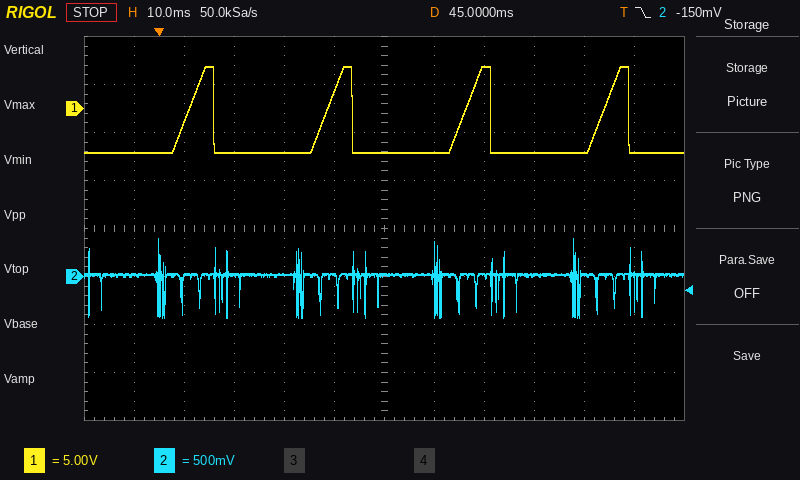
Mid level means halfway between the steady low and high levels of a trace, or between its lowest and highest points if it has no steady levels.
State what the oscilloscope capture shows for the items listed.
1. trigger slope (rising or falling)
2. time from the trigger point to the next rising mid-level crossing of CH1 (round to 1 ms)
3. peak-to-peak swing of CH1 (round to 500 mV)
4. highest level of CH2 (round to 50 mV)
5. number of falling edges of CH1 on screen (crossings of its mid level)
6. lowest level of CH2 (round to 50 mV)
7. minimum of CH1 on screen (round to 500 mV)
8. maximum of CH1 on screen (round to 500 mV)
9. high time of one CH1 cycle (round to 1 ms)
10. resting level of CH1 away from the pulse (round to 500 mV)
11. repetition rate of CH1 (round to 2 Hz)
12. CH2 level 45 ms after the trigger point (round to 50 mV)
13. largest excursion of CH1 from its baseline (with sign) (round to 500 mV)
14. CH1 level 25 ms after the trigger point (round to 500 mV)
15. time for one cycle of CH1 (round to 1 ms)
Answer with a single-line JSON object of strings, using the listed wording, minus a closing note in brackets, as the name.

{"trigger slope": "falling", "time from the trigger point to the next rising mid-level crossing of CH1": "6 ms", "peak-to-peak swing of CH1": "9.0 V", "highest level of CH2": "400 mV", "number of falling edges of CH1 on screen": "4", "lowest level of CH2": "-450 mV", "minimum of CH1 on screen": "-4.5 V", "maximum of CH1 on screen": "4.5 V", "high time of one CH1 cycle": "5 ms", "resting level of CH1 away from the pulse": "-4.5 V", "repetition rate of CH1": "36 Hz", "CH2 level 45 ms after the trigger point": "0 mV", "largest excursion of CH1 from its baseline (with sign)": "+9.0 V", "CH1 level 25 ms after the trigger point": "-4.5 V", "time for one cycle of CH1": "28 ms"}
